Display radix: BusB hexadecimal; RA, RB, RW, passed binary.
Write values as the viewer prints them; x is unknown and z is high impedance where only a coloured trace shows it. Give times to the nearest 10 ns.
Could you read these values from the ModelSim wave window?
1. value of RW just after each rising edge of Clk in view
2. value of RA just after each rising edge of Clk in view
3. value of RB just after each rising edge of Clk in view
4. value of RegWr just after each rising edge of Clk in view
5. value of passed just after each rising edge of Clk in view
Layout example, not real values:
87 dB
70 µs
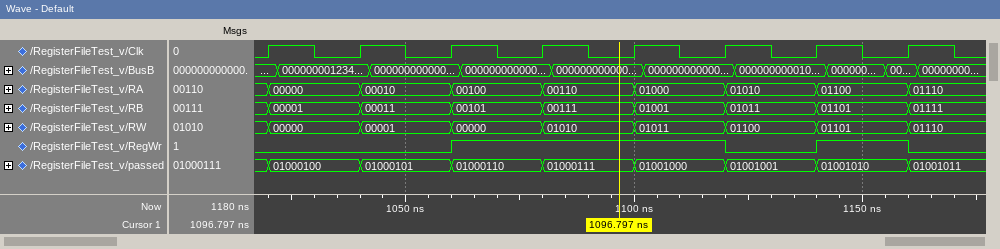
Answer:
00000, 00001, 00000, 01010, 01011, 01100, 01101, 01110
00000, 00010, 00100, 00110, 01000, 01010, 01100, 01110
00001, 00011, 00101, 00111, 01001, 01011, 01101, 01111
0 0 1 1 1 0 1 0
01000100, 01000101, 01000110, 01000111, 01001000, 01001001, 01001010, 01001011
